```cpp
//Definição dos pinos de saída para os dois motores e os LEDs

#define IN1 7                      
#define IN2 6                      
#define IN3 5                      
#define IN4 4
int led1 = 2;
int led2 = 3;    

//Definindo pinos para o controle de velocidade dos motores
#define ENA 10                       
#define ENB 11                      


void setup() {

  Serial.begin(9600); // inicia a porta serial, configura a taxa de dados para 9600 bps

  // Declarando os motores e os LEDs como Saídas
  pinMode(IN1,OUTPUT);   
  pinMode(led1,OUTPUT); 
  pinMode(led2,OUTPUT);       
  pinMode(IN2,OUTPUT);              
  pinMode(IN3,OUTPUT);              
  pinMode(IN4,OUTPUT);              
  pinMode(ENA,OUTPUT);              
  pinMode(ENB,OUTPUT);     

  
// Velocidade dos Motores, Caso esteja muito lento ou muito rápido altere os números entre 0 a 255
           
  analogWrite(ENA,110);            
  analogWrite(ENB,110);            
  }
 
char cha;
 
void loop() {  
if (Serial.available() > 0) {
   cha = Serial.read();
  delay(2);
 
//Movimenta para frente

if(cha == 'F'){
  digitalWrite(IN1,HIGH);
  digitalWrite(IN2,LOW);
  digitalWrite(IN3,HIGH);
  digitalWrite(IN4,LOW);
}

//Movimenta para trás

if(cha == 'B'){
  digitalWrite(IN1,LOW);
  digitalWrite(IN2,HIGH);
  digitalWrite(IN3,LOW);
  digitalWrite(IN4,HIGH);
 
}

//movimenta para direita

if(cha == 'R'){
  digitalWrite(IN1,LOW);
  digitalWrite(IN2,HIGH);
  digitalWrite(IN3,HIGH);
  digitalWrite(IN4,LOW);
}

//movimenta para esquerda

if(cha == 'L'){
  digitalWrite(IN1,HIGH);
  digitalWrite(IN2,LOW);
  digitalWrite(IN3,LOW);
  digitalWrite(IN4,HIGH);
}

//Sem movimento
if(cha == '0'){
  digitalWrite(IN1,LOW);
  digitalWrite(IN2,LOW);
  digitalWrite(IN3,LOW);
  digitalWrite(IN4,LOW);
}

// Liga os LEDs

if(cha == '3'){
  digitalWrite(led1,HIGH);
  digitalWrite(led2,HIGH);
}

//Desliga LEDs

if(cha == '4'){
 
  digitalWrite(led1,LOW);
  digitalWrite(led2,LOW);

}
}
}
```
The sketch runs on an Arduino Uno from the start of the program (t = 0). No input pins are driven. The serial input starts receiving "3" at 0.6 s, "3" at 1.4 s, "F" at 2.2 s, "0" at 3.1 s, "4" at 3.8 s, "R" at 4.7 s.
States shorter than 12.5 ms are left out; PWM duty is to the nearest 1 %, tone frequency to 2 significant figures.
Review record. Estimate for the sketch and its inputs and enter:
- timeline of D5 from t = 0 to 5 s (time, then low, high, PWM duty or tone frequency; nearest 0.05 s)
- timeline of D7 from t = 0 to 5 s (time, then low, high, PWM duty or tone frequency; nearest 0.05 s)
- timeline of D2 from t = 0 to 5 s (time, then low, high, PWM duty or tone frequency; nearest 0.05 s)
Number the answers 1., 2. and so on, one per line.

1. 0 s low; 2.2 s high; 3.1 s low; 4.7 s high
2. 0 s low; 2.2 s high; 3.1 s low
3. 0 s low; 0.6 s high; 3.8 s low
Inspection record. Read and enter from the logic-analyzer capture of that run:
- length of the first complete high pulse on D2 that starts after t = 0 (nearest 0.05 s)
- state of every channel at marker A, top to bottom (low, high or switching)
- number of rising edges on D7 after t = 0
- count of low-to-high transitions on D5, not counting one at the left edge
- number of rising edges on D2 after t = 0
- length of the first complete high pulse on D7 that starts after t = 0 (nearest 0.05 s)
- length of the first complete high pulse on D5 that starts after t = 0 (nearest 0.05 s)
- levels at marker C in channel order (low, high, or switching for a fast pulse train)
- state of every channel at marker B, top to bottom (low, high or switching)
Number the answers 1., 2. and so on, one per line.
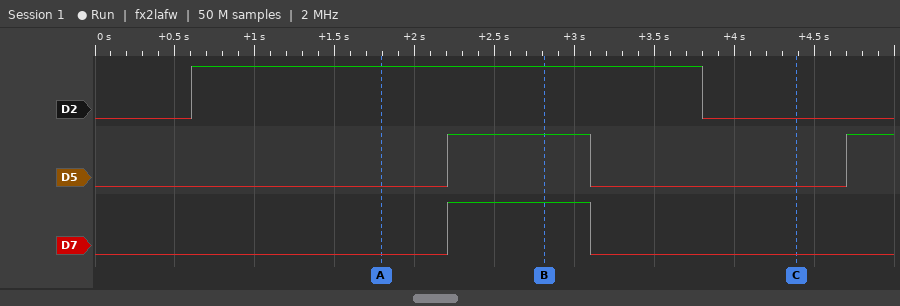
1. 3.20 s
2. D2 high, D5 low, D7 low
3. 1
4. 2
5. 1
6. 0.90 s
7. 0.90 s
8. D2 low, D5 low, D7 low
9. D2 high, D5 high, D7 high
